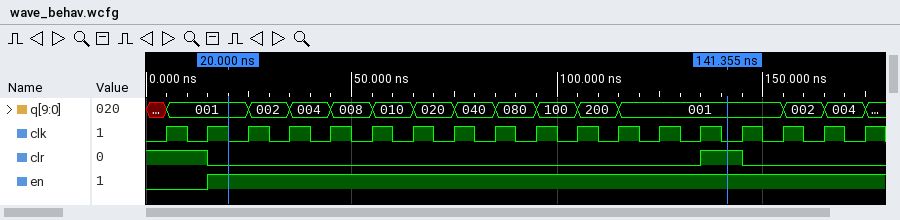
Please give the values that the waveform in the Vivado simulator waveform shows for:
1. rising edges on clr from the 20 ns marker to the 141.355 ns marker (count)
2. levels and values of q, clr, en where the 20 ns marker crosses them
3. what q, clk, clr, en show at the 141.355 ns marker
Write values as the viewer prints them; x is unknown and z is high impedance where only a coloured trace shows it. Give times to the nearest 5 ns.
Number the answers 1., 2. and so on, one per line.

1. 1
2. q=001, clr=0, en=1
3. q=001, clk=0, clr=1, en=1
